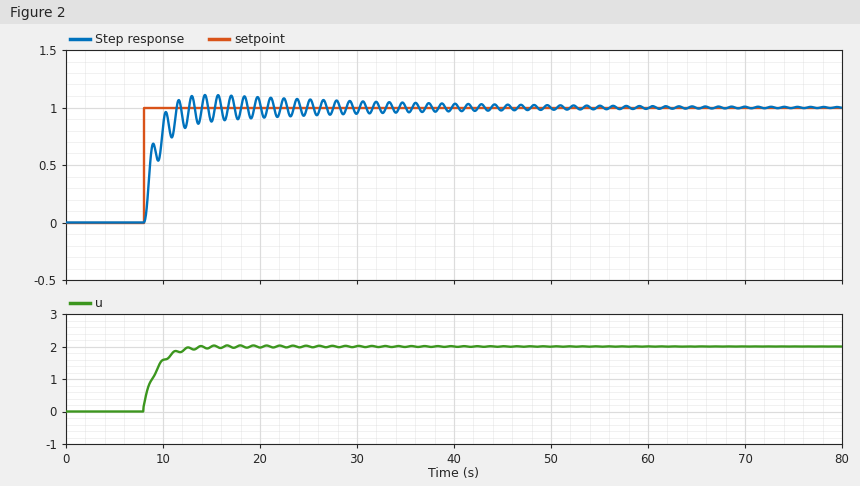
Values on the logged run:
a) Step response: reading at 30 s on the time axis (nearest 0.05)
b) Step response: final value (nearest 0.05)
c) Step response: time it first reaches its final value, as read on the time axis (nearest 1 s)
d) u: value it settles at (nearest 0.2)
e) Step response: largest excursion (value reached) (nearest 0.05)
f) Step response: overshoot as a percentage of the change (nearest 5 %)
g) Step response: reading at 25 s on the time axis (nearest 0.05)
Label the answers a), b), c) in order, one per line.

a) 0.95
b) 1.00
c) 11 s
d) 2.0
e) 1.10
f) 10 %
g) 1.05
